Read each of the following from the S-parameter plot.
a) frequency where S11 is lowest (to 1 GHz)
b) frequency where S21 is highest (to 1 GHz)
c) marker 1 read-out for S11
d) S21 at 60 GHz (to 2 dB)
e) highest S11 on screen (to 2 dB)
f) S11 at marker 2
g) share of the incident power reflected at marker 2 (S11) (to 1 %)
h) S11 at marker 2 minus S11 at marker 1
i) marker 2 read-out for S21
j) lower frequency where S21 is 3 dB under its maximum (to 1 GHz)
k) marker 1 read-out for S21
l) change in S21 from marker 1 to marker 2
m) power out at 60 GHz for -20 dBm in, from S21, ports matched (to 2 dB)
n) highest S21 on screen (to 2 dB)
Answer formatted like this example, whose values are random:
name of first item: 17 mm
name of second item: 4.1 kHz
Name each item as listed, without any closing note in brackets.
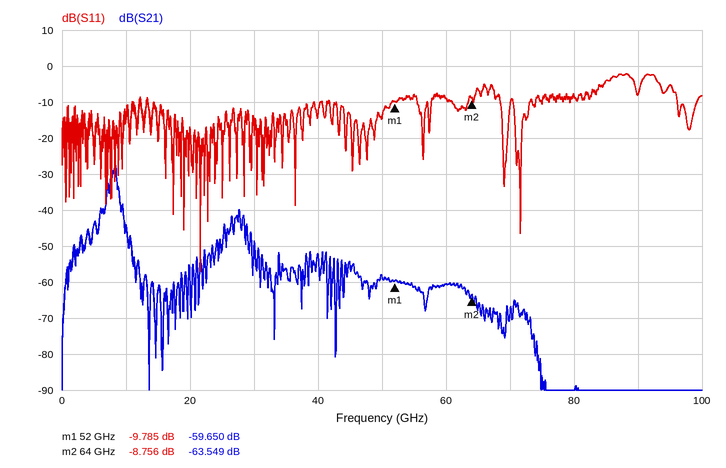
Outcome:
frequency where S11 is lowest: 22 GHz
frequency where S21 is highest: 8 GHz
marker 1 read-out for S11: -9.785 dB
S21 at 60 GHz: -60 dB
highest S11 on screen: -2 dB
S11 at marker 2: -8.756 dB
share of the incident power reflected at marker 2 (S11): 13 %
S11 at marker 2 minus S11 at marker 1: 1.029 dB
marker 2 read-out for S21: -63.549 dB
lower frequency where S21 is 3 dB under its maximum: 8 GHz
marker 1 read-out for S21: -59.650 dB
change in S21 from marker 1 to marker 2: -3.899 dB
power out at 60 GHz for -20 dBm in, from S21, ports matched: -80 dBm
highest S21 on screen: -28 dB
